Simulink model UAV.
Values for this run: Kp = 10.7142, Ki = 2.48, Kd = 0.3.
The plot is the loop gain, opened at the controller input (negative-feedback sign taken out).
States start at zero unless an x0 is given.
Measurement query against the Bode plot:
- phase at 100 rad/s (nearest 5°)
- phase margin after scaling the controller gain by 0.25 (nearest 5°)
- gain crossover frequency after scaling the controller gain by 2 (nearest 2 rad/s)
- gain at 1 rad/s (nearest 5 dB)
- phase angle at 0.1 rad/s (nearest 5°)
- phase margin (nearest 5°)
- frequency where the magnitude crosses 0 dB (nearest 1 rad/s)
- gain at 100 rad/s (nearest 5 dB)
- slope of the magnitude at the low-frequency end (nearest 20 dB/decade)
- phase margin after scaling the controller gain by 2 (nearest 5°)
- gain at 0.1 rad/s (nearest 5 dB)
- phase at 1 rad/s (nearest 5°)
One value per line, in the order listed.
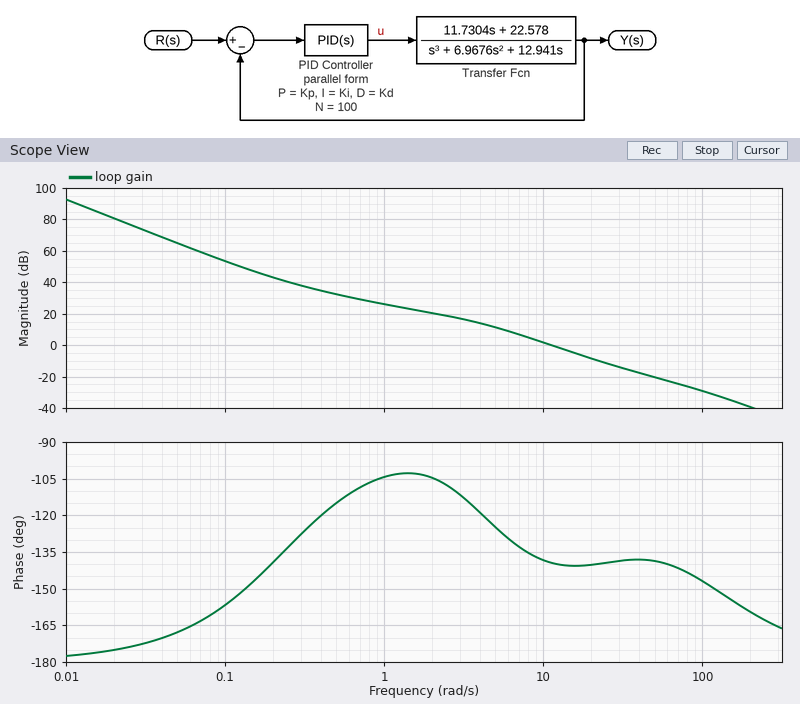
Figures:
-145°
55°
16 rad/s
25 dB
-155°
40°
11 rad/s
-30 dB
-40 dB/decade
40°
55 dB
-105°
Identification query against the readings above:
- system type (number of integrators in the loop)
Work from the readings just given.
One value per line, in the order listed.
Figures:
2
